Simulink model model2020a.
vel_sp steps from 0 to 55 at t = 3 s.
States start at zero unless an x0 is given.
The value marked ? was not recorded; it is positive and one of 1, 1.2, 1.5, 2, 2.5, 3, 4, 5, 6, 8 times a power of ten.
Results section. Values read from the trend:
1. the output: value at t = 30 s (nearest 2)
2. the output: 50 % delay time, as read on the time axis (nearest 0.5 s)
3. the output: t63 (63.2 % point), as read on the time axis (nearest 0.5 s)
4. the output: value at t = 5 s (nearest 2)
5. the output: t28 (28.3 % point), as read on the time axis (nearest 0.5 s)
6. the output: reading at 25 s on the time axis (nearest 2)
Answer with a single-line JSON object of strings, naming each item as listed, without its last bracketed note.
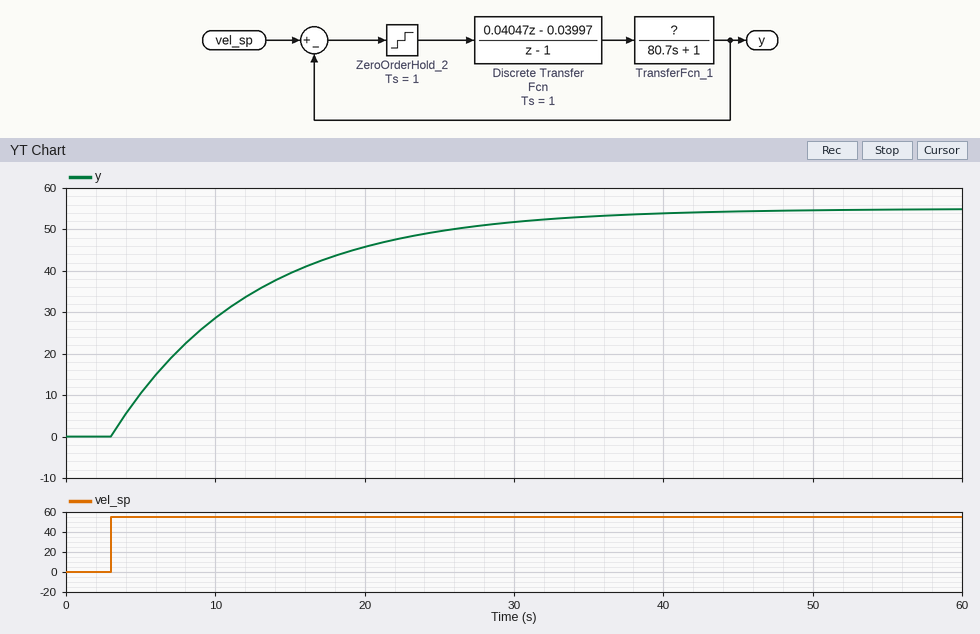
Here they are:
{"the output: value at t = 30 s": "52", "the output: 50 % delay time, as read on the time axis": "9.5 s", "the output: t63 (63.2 % point), as read on the time axis": "12.5 s", "the output: value at t = 5 s": "10", "the output: t28 (28.3 % point), as read on the time axis": "6.0 s", "the output: reading at 25 s on the time axis": "50"}
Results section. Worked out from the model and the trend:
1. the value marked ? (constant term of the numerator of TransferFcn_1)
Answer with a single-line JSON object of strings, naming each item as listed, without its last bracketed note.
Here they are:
{"the value marked ?": "200"}
